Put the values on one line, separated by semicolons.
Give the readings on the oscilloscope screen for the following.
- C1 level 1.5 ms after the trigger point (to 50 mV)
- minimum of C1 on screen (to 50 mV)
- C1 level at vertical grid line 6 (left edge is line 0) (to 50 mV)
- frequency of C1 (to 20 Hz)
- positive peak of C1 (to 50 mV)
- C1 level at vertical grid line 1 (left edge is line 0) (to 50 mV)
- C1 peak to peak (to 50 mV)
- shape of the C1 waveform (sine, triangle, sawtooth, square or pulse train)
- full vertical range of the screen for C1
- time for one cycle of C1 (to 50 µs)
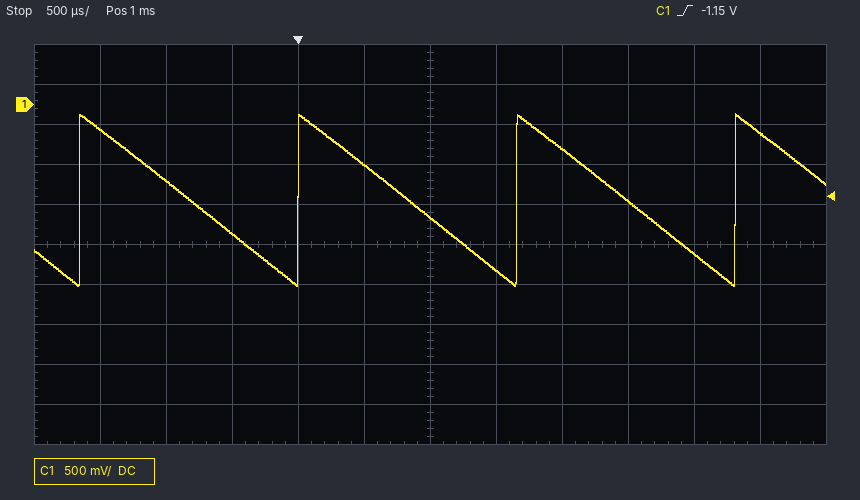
-2.05 V; -2.25 V; -1.40 V; 600 Hz; -100 mV; -300 mV; 2.15 V; sawtooth; 5 V; 1.65 ms
